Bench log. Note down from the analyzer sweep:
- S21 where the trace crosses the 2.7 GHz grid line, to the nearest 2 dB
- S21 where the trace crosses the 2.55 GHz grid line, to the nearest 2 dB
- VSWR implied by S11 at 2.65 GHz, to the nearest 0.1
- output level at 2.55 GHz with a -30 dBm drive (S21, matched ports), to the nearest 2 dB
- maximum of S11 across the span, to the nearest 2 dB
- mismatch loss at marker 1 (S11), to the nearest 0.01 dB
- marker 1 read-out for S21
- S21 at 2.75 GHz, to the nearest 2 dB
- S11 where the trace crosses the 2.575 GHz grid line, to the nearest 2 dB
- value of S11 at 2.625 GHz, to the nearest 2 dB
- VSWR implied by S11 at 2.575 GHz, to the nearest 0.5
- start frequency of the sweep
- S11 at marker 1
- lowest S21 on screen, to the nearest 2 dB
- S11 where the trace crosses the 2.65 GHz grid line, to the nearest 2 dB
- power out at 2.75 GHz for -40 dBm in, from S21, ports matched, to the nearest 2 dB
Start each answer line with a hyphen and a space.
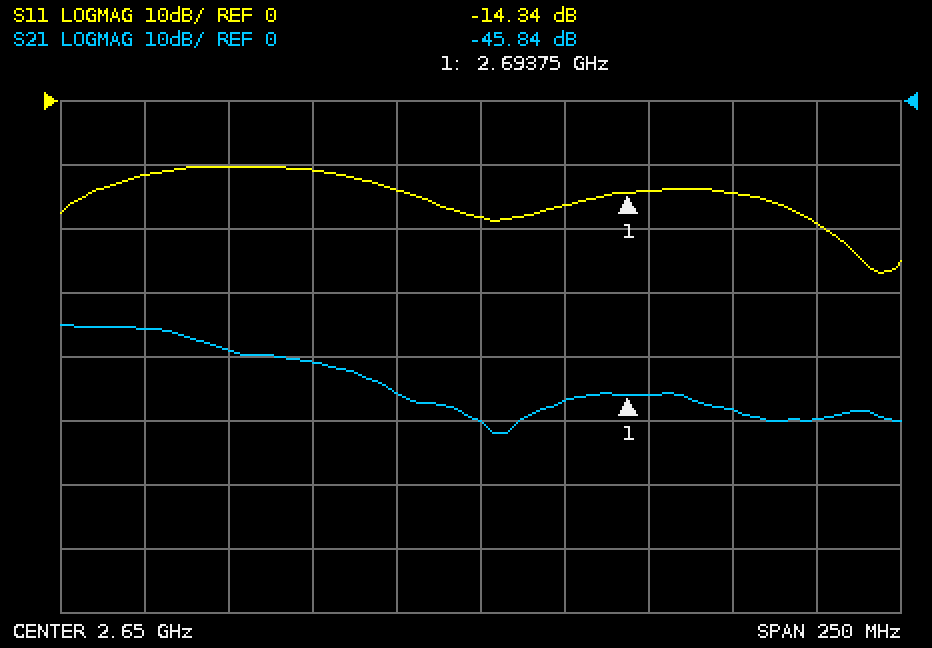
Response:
- -46 dB
- -36 dB
- 1.3
- -66 dBm
- -10 dB
- 0.16 dB
- -45.84 dB
- -50 dB
- -10 dB
- -14 dB
- 2.0
- 2.525 GHz
- -14.34 dB
- -52 dB
- -18 dB
- -90 dBm
